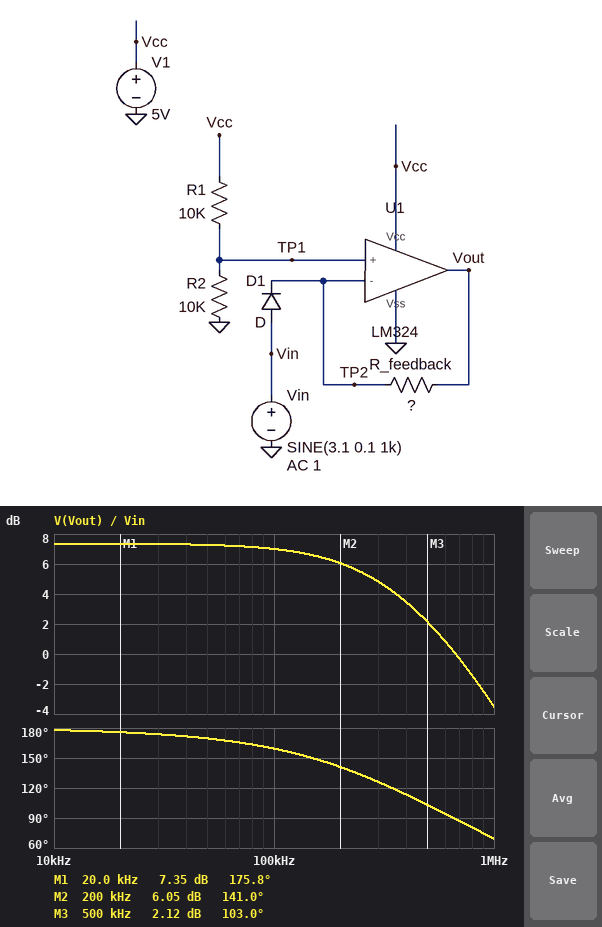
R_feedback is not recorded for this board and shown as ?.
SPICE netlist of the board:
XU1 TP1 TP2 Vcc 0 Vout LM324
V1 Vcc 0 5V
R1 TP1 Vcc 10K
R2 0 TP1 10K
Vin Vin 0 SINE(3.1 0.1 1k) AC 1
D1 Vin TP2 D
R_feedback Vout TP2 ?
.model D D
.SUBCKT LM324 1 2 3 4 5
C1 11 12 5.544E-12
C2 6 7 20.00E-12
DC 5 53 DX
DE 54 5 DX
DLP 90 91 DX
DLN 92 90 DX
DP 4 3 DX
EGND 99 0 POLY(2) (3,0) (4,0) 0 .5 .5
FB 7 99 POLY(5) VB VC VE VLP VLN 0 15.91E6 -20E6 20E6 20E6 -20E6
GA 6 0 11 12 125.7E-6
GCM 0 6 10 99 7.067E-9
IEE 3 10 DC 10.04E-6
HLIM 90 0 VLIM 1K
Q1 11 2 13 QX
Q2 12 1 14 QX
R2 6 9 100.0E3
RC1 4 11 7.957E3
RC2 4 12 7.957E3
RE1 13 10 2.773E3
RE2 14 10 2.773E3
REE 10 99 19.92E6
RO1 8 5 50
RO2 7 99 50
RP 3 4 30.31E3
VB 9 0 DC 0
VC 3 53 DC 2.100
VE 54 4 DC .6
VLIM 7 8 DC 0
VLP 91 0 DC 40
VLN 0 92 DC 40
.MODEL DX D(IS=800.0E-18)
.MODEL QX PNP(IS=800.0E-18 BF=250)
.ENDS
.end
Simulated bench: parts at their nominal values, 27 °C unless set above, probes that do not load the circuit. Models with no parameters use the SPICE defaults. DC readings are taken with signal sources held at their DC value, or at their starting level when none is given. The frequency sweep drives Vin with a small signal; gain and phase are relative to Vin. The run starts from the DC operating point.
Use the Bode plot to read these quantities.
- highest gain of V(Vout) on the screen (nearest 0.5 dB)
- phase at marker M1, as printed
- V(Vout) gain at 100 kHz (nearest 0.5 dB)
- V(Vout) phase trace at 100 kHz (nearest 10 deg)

7.5 dB
175.8 deg
7.0 dB
160 deg
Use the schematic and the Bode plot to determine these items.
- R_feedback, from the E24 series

510 Ω
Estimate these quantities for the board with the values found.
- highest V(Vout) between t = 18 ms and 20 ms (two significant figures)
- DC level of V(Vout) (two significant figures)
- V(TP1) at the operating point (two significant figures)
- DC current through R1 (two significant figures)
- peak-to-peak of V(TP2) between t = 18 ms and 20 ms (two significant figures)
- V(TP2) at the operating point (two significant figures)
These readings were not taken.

2.5 V
2.4 V
2.5 V
250 µA
8.4 mV
2.5 V
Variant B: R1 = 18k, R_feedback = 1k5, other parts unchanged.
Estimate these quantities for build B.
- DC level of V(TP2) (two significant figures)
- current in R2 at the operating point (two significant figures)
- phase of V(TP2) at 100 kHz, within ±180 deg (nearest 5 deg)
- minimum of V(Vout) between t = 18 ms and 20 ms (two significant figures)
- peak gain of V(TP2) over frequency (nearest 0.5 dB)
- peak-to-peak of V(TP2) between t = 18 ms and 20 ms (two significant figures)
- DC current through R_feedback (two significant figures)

2.4 V
180 µA
0 deg
4.6 mV
0 dB
200 mV
1.6 mA
